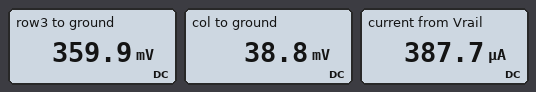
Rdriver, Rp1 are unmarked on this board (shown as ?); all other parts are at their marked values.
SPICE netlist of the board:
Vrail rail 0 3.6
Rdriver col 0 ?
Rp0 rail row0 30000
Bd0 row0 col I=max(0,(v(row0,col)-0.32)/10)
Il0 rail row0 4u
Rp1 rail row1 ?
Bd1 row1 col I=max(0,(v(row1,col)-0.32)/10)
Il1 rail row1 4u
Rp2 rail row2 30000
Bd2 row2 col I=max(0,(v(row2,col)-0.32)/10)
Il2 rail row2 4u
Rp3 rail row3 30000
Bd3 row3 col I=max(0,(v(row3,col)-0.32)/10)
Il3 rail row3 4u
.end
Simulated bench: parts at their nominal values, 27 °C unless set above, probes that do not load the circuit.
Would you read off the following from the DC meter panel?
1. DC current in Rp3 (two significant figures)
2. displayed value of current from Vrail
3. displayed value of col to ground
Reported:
110 µA
387.7 µA
38.8 mV
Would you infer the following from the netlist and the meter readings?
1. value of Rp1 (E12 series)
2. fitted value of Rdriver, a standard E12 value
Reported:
68 kΩ
100 Ω
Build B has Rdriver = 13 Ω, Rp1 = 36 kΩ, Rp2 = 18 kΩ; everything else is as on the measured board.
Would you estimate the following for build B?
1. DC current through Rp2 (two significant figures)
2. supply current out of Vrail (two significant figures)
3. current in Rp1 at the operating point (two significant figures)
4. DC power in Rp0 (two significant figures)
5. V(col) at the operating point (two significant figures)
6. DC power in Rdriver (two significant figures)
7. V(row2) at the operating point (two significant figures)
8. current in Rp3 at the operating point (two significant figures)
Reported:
180 µA
510 µA
91 µA
360 µW
6.6 mV
3.3 µW
330 mV
110 µA
